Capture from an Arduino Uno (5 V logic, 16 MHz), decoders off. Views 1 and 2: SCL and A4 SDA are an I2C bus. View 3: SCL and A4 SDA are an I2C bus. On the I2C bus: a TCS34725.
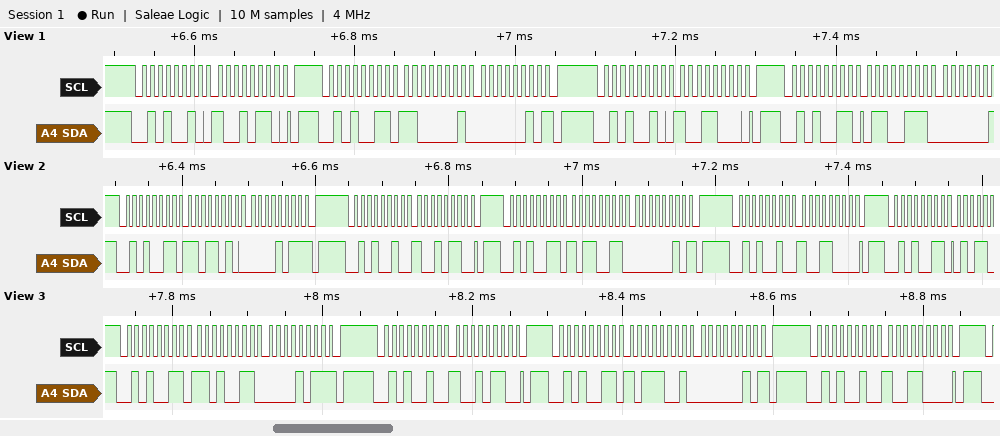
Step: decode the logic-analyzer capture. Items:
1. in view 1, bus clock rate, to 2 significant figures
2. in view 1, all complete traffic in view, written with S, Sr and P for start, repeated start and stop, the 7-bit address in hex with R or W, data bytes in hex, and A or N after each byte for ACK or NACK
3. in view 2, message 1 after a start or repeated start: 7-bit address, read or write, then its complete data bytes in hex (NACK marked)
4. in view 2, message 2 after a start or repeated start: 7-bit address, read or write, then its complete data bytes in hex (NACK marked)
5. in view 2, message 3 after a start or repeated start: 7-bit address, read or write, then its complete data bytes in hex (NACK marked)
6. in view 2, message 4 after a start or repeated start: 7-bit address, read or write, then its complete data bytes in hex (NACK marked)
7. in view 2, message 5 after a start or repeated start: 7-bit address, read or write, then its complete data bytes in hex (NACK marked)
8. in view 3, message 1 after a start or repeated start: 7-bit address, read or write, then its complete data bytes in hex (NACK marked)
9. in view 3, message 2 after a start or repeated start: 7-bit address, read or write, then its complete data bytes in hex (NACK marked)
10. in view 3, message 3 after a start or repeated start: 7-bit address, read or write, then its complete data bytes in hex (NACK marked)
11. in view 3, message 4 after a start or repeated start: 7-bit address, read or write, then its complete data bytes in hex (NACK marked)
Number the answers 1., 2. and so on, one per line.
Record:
1. 100 kHz
2. S 29W A 96 A P S 29R A C1 A 02 N P S 29W A 98 A P S 29R A 67 A
3. 0x29 read: DA 0B NACK
4. 0x29 write: 96
5. 0x29 read: B3 02 NACK
6. 0x29 write: 98
7. 0x29 read
8. 0x29 read: D3 0B NACK
9. 0x29 write: 96
10. 0x29 read: B9 02 NACK
11. 0x29 write: 98
